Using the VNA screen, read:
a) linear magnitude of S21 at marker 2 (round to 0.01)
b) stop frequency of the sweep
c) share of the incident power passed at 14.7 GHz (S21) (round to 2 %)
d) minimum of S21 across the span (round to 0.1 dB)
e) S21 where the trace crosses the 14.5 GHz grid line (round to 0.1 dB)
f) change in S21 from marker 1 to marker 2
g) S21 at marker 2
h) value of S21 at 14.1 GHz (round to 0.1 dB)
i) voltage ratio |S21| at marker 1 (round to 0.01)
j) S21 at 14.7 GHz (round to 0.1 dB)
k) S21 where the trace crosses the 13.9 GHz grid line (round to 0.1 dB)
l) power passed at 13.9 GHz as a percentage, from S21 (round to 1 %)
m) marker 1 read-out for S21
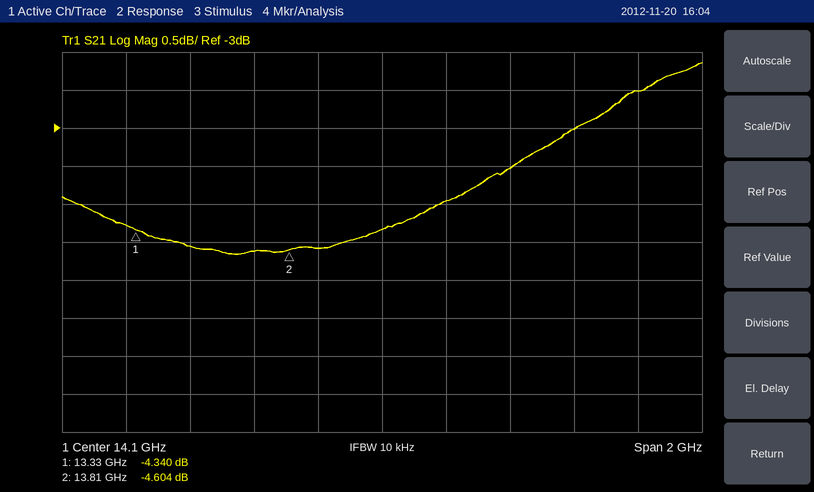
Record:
0.59
15.1 GHz
50 %
-4.7 dB
-3.5 dB
-0.264 dB
-4.604 dB
-4.3 dB
0.61
-3.0 dB
-4.6 dB
35 %
-4.340 dB
